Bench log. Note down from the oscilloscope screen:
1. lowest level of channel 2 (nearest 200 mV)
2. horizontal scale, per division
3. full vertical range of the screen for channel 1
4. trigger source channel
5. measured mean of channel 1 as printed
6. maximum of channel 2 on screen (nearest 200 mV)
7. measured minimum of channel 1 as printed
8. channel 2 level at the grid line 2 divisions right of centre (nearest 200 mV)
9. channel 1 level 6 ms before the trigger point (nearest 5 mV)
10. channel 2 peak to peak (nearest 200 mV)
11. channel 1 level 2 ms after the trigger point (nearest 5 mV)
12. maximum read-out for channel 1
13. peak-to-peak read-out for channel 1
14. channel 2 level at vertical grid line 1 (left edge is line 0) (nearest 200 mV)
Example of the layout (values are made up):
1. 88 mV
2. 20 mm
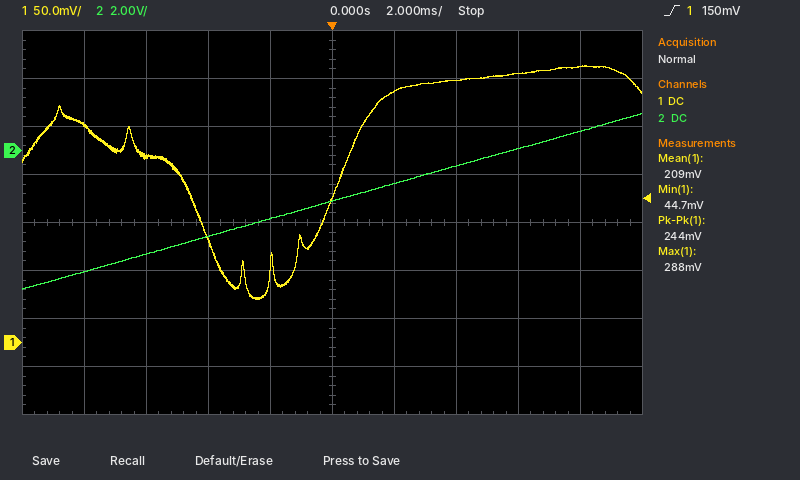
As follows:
1. -5.8 V
2. 2 ms
3. 400 mV
4. channel 1
5. 209 mV
6. 1.6 V
7. 44.7 mV
8. -600 mV
9. 195 mV
10. 7.4 V
11. 260 mV
12. 288 mV
13. 244 mV
14. -5.0 V
